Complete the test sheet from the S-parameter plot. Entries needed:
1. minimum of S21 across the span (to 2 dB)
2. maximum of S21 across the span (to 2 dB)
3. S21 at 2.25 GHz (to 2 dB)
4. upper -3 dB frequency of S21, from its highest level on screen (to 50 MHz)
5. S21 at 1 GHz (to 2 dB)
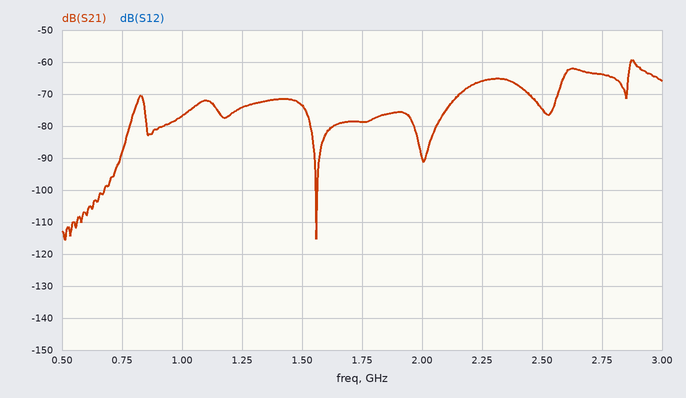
-116 dB
-60 dB
-66 dB
2.90 GHz
-76 dB
